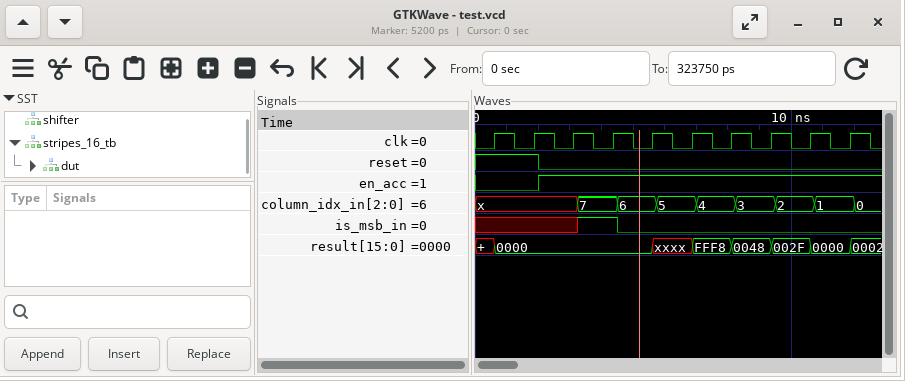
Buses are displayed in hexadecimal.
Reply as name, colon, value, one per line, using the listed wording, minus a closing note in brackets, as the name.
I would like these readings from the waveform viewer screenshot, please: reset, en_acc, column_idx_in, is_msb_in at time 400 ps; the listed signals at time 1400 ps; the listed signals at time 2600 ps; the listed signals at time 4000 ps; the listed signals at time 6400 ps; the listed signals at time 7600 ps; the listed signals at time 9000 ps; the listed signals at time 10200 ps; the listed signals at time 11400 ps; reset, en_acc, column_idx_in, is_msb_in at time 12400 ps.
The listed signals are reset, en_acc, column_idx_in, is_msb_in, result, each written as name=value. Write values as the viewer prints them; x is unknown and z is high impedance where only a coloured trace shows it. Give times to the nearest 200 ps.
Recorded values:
reset, en_acc, column_idx_in, is_msb_in at time 400 ps: reset=1, en_acc=0, column_idx_in=x, is_msb_in=x
the listed signals at time 1400 ps: reset=1, en_acc=0, column_idx_in=x, is_msb_in=x, result=0000
the listed signals at time 2600 ps: reset=0, en_acc=1, column_idx_in=x, is_msb_in=x, result=0000
the listed signals at time 4000 ps: reset=0, en_acc=1, column_idx_in=7, is_msb_in=1, result=0000
the listed signals at time 6400 ps: reset=0, en_acc=1, column_idx_in=5, is_msb_in=0, result=xxxx
the listed signals at time 7600 ps: reset=0, en_acc=1, column_idx_in=4, is_msb_in=0, result=FFF8
the listed signals at time 9000 ps: reset=0, en_acc=1, column_idx_in=3, is_msb_in=0, result=0048
the listed signals at time 10200 ps: reset=0, en_acc=1, column_idx_in=2, is_msb_in=0, result=002F
the listed signals at time 11400 ps: reset=0, en_acc=1, column_idx_in=1, is_msb_in=0, result=0000
reset, en_acc, column_idx_in, is_msb_in at time 12400 ps: reset=0, en_acc=1, column_idx_in=0, is_msb_in=0
